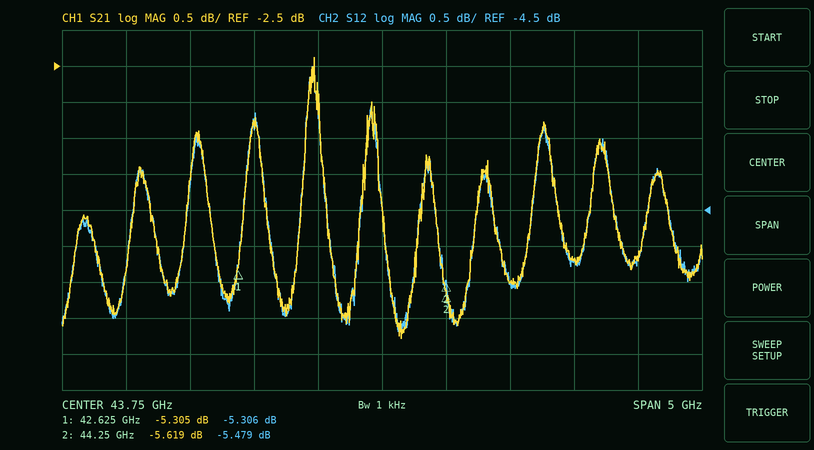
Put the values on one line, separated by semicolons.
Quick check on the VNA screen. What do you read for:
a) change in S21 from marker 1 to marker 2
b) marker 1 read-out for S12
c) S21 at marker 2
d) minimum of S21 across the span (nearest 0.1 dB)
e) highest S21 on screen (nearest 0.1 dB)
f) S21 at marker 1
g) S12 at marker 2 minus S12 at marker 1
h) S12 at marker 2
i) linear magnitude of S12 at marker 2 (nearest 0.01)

-0.314 dB; -5.306 dB; -5.619 dB; -6.3 dB; -2.4 dB; -5.305 dB; -0.173 dB; -5.479 dB; 0.53
